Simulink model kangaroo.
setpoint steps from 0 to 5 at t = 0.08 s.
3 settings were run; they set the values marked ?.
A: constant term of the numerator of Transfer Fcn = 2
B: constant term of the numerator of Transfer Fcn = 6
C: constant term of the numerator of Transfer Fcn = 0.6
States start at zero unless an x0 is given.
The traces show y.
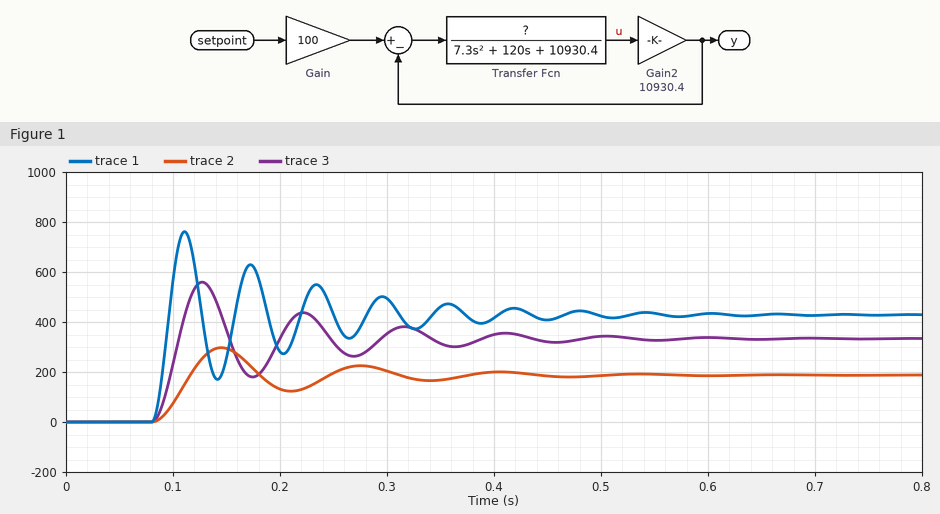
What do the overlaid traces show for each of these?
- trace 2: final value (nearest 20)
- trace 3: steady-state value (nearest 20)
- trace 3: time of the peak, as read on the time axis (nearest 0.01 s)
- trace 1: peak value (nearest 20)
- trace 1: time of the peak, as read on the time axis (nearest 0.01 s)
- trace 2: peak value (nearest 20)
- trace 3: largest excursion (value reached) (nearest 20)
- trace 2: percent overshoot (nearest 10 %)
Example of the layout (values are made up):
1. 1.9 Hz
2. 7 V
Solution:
1. 180
2. 340
3. 0.13 s
4. 760
5. 0.11 s
6. 300
7. 560
8. 60 %
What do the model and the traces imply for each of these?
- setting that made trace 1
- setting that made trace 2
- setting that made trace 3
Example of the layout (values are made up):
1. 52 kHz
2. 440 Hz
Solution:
1. B
2. C
3. A
